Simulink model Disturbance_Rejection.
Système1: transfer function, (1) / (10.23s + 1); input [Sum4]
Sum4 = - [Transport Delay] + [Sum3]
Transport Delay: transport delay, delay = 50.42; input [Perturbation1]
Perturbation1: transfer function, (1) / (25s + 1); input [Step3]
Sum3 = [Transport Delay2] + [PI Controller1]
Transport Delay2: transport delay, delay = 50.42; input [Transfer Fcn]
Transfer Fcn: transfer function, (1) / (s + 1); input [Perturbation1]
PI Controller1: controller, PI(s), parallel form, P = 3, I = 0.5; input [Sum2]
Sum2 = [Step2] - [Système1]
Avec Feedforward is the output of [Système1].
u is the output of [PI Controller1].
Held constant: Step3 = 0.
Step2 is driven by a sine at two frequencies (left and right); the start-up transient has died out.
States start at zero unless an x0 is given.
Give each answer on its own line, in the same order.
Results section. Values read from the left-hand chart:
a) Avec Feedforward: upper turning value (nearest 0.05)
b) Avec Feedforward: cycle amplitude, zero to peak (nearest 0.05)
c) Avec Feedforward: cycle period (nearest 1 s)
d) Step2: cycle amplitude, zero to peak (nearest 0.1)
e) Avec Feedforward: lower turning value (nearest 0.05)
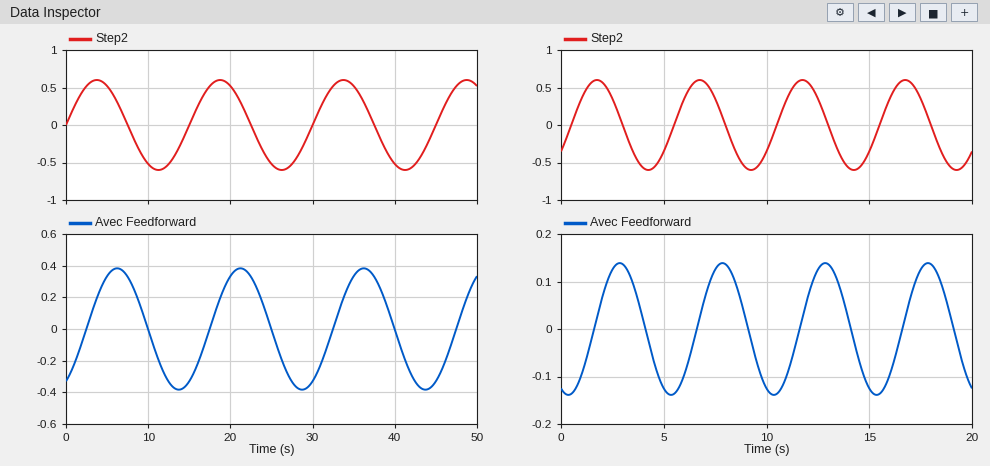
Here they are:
0.40
0.40
15 s
0.6
-0.40
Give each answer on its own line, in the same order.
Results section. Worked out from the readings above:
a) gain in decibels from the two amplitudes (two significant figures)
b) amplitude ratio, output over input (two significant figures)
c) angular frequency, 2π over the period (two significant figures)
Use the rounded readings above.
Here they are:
-3.5 dB
0.67
0.42 rad/s
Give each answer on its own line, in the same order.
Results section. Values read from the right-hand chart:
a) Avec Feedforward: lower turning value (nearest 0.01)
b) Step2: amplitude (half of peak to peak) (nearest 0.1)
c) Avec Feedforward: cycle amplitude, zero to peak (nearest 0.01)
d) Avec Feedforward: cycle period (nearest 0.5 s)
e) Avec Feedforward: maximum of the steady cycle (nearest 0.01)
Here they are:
-0.14
0.6
0.14
5.0 s
0.14
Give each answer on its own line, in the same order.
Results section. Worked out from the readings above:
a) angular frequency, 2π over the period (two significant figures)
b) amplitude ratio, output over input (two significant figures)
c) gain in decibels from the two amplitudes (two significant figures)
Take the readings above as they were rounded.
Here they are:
1.3 rad/s
0.23
-13 dB
